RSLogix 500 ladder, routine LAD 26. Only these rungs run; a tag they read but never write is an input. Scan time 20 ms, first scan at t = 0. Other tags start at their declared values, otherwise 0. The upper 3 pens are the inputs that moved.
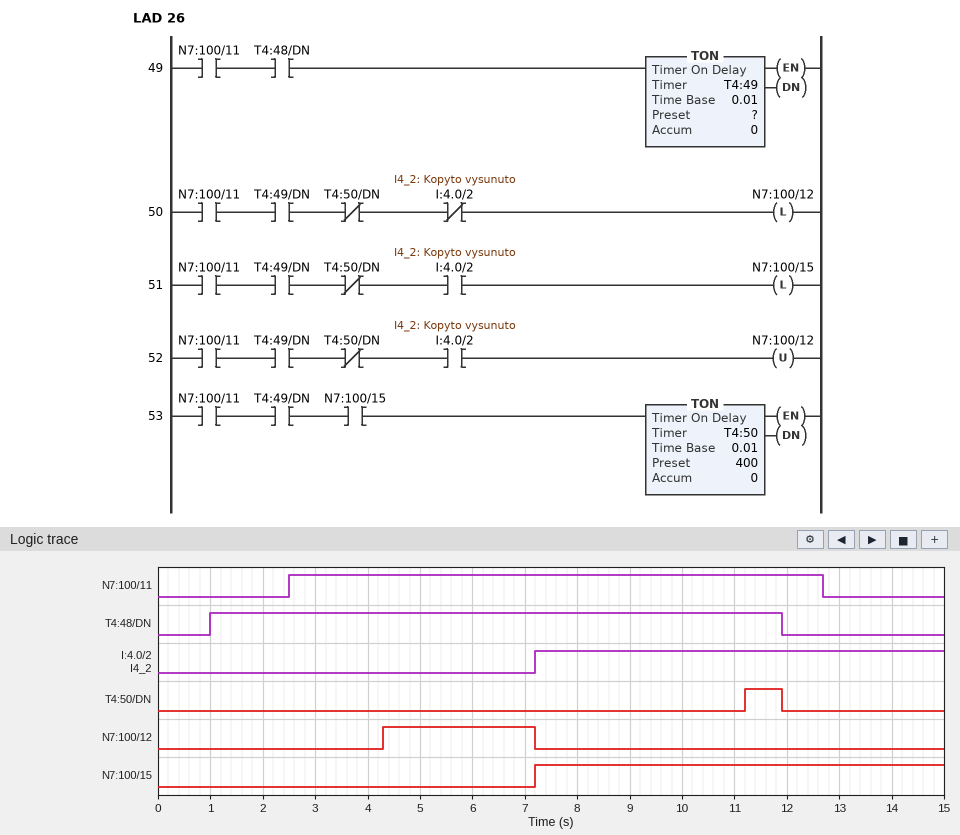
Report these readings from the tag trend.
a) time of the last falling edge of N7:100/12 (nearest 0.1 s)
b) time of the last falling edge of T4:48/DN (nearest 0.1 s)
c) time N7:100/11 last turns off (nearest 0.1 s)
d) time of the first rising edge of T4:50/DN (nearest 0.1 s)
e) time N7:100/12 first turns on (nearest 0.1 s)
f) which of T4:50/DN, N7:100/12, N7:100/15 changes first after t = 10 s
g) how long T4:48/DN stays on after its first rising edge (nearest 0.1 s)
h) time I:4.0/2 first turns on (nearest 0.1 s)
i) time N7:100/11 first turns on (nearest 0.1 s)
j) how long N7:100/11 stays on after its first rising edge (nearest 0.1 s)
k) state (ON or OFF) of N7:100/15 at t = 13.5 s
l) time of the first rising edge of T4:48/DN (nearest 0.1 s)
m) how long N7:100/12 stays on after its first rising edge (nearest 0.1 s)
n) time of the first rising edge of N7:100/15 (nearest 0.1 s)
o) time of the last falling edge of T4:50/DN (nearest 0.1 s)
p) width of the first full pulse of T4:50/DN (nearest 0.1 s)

7.2 s
11.9 s
12.7 s
11.2 s
4.3 s
T4:50/DN
10.9 s
7.2 s
2.5 s
10.2 s
ON
1.0 s
2.9 s
7.2 s
11.9 s
0.7 s
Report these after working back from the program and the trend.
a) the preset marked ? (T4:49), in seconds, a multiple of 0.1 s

1.8 s
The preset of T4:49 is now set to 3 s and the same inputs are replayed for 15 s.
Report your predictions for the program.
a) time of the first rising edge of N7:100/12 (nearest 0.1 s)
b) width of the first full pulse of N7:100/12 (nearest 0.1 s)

5.5 s
1.7 s
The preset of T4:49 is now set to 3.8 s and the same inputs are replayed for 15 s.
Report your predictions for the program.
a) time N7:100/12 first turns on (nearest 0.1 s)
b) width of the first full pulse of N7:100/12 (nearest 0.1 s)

6.3 s
0.9 s
